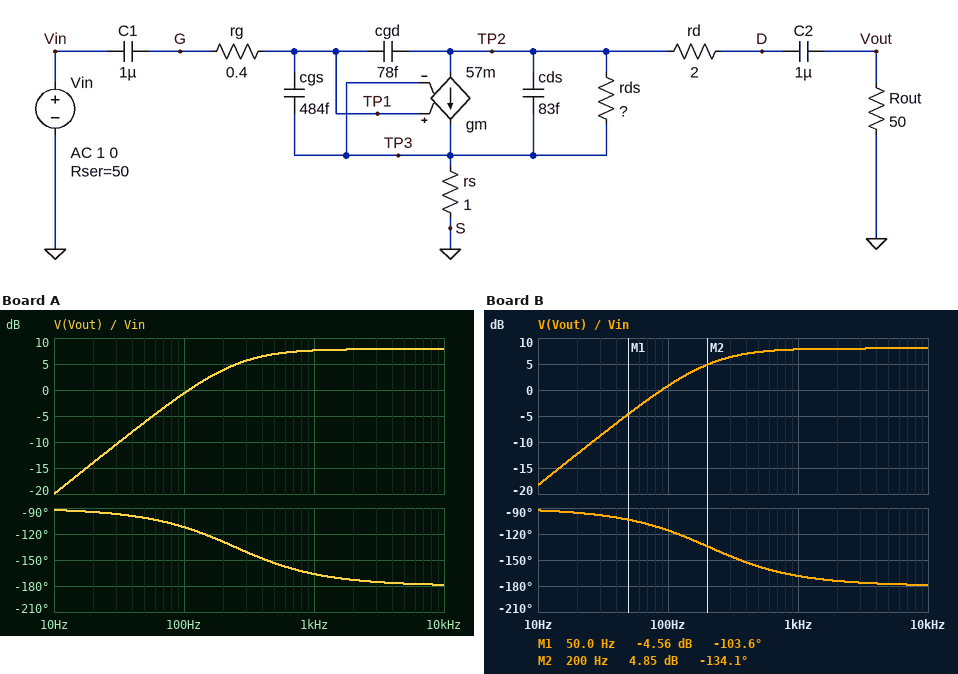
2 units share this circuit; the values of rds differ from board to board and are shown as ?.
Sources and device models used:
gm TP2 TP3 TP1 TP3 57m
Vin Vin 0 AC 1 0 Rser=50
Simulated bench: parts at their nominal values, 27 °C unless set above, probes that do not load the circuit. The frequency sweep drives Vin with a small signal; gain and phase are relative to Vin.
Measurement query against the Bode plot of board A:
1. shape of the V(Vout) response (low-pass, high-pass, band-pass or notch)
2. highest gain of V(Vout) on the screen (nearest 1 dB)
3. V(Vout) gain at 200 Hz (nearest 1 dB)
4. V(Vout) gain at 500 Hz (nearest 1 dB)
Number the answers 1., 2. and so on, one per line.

1. high-pass
2. 8 dB
3. 4 dB
4. 7 dB
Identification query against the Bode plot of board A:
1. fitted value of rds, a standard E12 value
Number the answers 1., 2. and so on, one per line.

1. 560 Ω
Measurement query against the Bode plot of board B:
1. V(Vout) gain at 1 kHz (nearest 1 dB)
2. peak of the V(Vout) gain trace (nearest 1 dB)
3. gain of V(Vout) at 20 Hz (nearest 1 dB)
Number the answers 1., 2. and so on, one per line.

1. 8 dB
2. 8 dB
3. -12 dB
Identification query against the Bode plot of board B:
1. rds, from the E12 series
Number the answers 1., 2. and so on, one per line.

1. 680 Ω
